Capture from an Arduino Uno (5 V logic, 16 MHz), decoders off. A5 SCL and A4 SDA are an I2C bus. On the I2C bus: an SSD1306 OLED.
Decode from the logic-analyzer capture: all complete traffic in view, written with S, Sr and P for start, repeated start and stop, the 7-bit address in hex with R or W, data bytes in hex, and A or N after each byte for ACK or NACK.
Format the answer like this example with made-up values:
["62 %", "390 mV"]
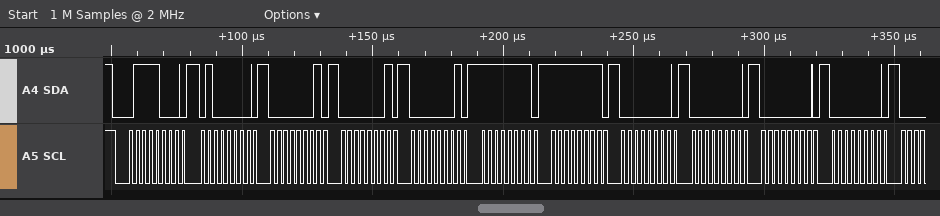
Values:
["S 3CW A 40 A 01 A 01 A 01 A FF A FF A 00 A 00 A 00 A 00 A"]
